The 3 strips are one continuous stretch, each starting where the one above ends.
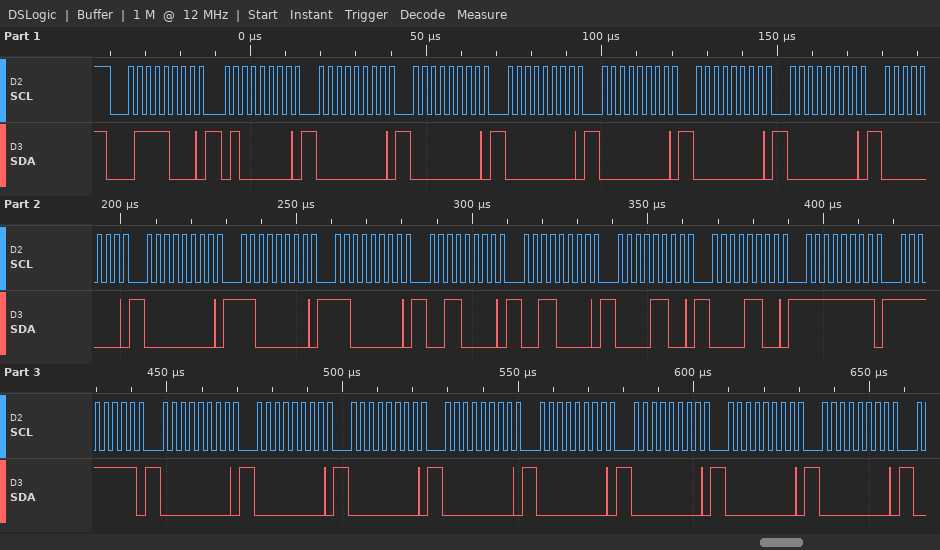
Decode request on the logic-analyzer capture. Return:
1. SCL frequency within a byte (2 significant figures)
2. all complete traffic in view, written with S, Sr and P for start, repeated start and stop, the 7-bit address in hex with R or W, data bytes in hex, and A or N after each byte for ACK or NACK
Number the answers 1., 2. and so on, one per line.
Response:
1. 400 kHz
2. S 3CW A 40 A 00 A 00 A 00 A 00 A 00 A 00 A 00 A 00 A C0 A C0 A 30 A 30 A 0C A 0C A FF A FF A 00 A 00 A 00 A 00 A 00 A 00 A 00 A 00 A
